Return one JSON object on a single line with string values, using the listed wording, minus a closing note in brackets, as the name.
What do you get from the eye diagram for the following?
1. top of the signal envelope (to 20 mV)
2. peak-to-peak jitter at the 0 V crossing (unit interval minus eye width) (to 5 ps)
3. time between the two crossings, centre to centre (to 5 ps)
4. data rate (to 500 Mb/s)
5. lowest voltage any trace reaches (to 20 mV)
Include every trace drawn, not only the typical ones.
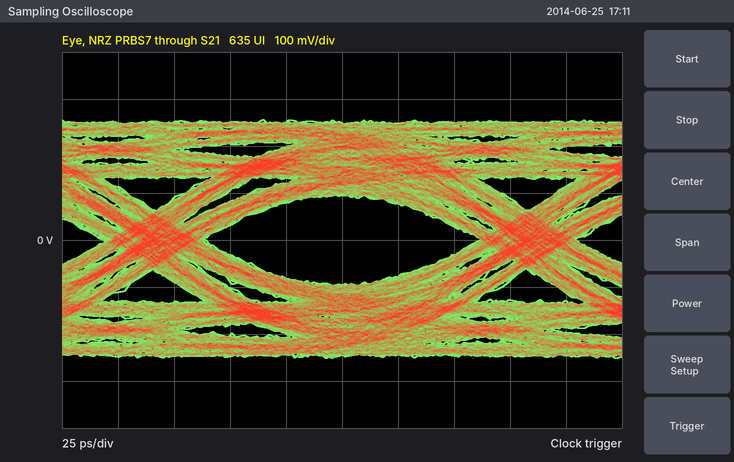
{"top of the signal envelope": "260 mV", "peak-to-peak jitter at the 0 V crossing (unit interval minus eye width)": "45 ps", "time between the two crossings, centre to centre": "165 ps", "data rate": "6.0 Gb/s", "lowest voltage any trace reaches": "-260 mV"}
